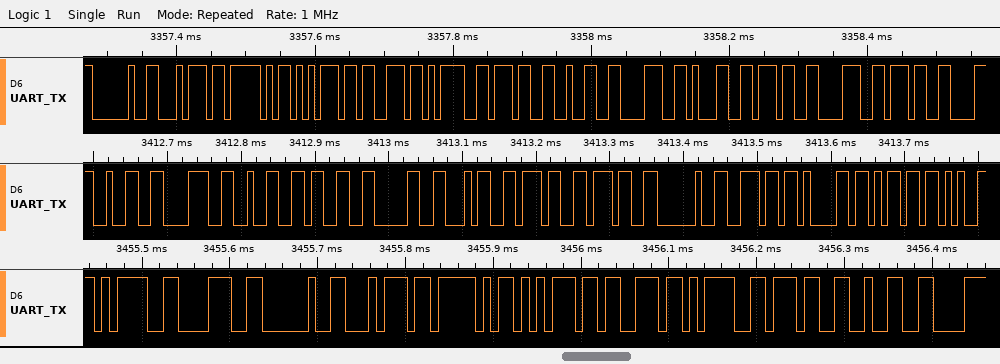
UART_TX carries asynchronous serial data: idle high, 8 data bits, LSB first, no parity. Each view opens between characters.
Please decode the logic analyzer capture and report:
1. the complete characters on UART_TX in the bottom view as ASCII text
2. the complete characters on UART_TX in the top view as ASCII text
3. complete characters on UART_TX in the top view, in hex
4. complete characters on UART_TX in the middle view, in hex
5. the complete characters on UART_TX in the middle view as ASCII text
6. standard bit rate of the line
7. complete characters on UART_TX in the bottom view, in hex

"=8 t_us=72"
" t_us=7281787"
20, 74, 5F, 75, 73, 3D, 37, 32, 38, 31, 37, 38, 37
32, 38, 32, 33, 30, 34, 37, 37, 20, 6E, 61, 6D
"28230477 nam"
115200 baud
3D, 38, 20, 74, 5F, 75, 73, 3D, 37, 32
